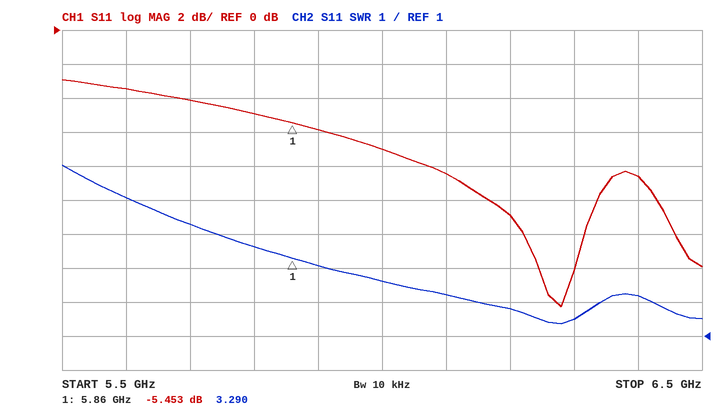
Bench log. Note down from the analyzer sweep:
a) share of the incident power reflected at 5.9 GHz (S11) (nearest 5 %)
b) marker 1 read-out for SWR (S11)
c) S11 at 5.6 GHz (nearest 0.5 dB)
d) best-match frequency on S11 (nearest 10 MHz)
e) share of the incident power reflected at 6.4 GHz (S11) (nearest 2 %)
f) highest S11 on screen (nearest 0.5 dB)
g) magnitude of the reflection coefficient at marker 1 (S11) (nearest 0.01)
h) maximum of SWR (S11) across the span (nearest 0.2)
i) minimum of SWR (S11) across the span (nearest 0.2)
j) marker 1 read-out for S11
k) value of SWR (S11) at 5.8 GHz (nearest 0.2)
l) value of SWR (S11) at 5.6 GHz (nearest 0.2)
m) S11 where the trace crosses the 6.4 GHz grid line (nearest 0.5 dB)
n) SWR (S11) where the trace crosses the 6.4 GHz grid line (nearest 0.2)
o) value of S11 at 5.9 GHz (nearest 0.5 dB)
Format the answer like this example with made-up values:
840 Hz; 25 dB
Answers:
25 %; 3.290; -3.5 dB; 6.28 GHz; 14 %; -3.0 dB; 0.53; 6.0; 1.4; -5.453 dB; 3.6; 5.0; -8.5 dB; 2.2; -6.0 dB
